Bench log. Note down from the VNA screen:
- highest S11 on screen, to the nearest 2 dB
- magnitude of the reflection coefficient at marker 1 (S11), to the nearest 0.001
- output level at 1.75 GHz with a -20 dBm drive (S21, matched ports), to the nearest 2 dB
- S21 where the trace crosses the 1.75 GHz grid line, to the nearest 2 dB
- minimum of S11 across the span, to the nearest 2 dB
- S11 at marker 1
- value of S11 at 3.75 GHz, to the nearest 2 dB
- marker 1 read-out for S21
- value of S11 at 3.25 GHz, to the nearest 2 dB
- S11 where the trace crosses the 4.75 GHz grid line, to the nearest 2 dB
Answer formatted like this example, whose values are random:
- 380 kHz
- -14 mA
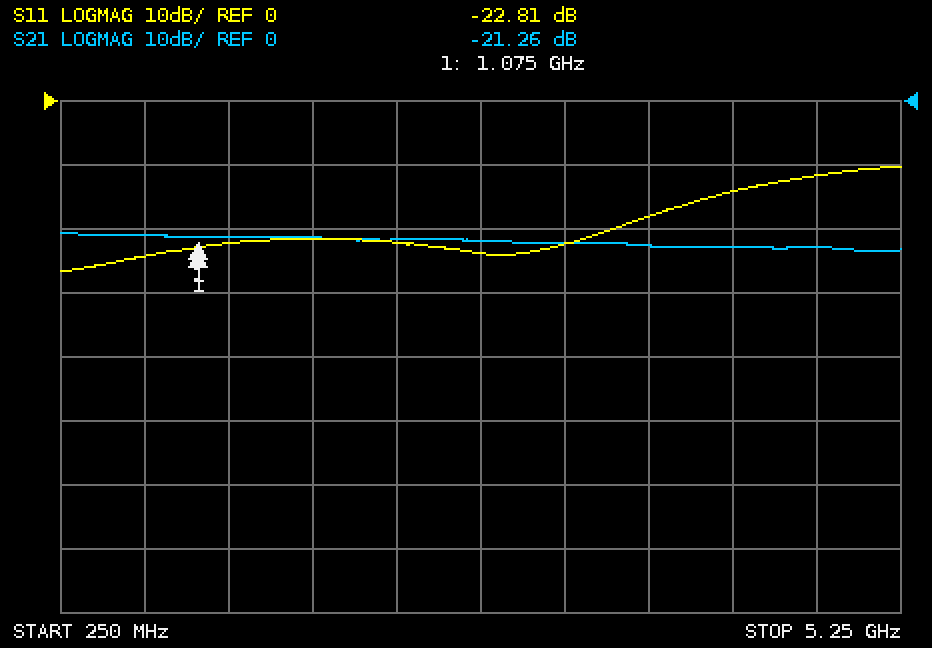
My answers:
- -10 dB
- 0.072
- -42 dBm
- -22 dB
- -26 dB
- -22.81 dB
- -18 dB
- -21.26 dB
- -22 dB
- -12 dB
